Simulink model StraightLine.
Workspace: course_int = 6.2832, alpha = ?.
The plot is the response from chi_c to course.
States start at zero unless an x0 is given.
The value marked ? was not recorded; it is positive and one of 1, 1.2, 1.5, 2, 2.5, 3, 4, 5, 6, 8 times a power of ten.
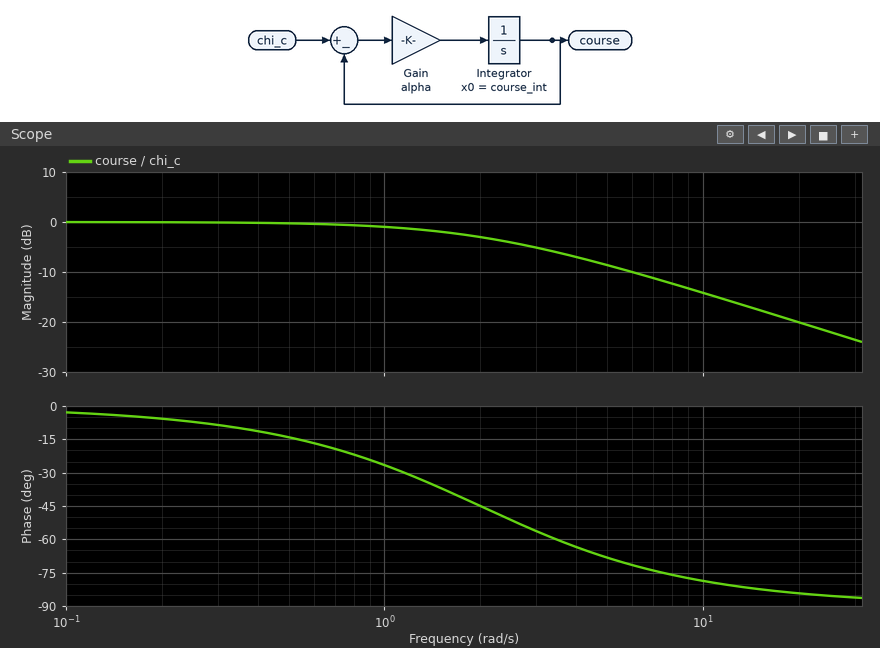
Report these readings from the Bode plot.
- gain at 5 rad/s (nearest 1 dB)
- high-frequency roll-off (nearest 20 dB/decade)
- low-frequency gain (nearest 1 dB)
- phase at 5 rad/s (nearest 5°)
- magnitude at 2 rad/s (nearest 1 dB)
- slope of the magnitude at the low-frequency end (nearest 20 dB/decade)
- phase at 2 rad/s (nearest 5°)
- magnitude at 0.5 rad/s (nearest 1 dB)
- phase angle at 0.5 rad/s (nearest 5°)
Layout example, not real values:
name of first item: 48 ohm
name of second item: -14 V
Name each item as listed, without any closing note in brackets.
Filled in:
gain at 5 rad/s: -9 dB
high-frequency roll-off: -20 dB/decade
low-frequency gain: 0 dB
phase at 5 rad/s: -70°
magnitude at 2 rad/s: -3 dB
slope of the magnitude at the low-frequency end: 0 dB/decade
phase at 2 rad/s: -45°
magnitude at 0.5 rad/s: 0 dB
phase angle at 0.5 rad/s: -15°
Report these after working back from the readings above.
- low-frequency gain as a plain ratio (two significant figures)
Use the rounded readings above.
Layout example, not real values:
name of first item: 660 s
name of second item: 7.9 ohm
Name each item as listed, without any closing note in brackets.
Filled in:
low-frequency gain as a plain ratio: 1.0
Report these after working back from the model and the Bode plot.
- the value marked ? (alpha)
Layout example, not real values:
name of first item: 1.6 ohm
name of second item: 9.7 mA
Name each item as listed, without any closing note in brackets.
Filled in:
the value marked ?: 2
